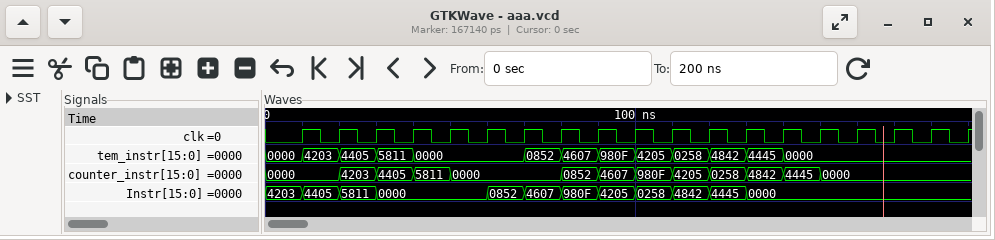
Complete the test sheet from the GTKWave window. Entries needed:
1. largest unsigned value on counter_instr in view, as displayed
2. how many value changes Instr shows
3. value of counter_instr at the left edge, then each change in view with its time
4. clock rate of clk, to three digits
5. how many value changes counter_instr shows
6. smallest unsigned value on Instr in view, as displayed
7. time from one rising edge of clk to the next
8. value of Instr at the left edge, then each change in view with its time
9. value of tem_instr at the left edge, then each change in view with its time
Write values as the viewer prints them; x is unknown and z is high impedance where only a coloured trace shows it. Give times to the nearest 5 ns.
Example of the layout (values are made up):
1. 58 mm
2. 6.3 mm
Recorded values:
1. 980F
2. 11
3. 0000, 4203 at 20 ns, 4405 at 30 ns, 5811 at 40 ns, 0000 at 50 ns, 0852 at 80 ns, 4607 at 90 ns, 980F at 100 ns, 4205 at 110 ns, 0258 at 120 ns, 4842 at 130 ns, 4445 at 140 ns, 0000 at 150 ns
4. 100 MHz
5. 12
6. 0000
7. 10 ns
8. 4203, 4405 at 10 ns, 5811 at 20 ns, 0000 at 30 ns, 0852 at 60 ns, 4607 at 70 ns, 980F at 80 ns, 4205 at 90 ns, 0258 at 100 ns, 4842 at 110 ns, 4445 at 120 ns, 0000 at 130 ns
9. 0000, 4203 at 10 ns, 4405 at 20 ns, 5811 at 30 ns, 0000 at 40 ns, 0852 at 70 ns, 4607 at 80 ns, 980F at 90 ns, 4205 at 100 ns, 0258 at 110 ns, 4842 at 120 ns, 4445 at 130 ns, 0000 at 140 ns
